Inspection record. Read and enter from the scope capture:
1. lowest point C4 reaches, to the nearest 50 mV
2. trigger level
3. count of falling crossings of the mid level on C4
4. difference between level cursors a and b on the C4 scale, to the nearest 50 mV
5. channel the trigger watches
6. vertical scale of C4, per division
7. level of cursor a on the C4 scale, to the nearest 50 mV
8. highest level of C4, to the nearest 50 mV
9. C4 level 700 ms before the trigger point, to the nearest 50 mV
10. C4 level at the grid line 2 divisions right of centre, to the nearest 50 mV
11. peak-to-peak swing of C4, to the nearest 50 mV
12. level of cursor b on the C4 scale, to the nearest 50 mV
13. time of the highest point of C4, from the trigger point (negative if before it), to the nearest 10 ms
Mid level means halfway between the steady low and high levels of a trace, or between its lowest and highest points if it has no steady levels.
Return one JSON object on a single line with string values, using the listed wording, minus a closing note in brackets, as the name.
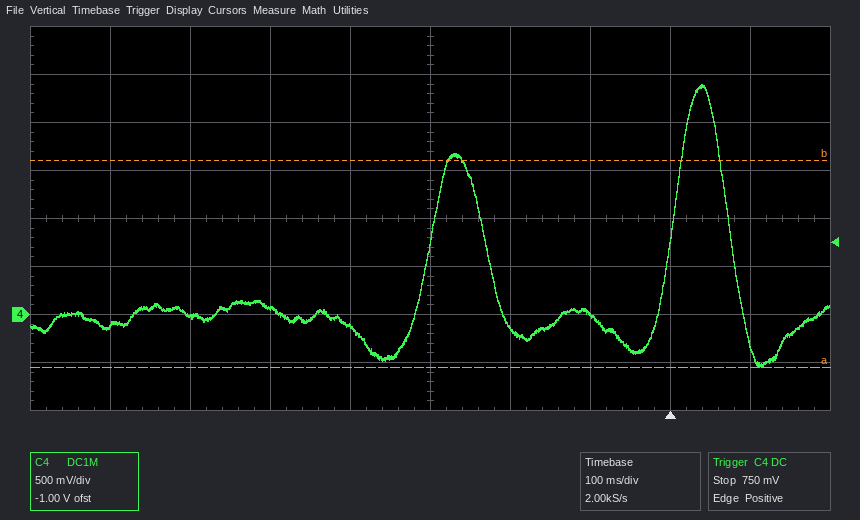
{"lowest point C4 reaches, to the nearest 50 mV": "-550 mV", "trigger level": "750 mV", "count of falling crossings of the mid level on C4": "2", "difference between level cursors a and b on the C4 scale, to the nearest 50 mV": "2.15 V", "channel the trigger watches": "C4", "vertical scale of C4, per division": "500 mV", "level of cursor a on the C4 scale, to the nearest 50 mV": "-550 mV", "highest level of C4, to the nearest 50 mV": "2.40 V", "C4 level 700 ms before the trigger point, to the nearest 50 mV": "-100 mV", "C4 level at the grid line 2 divisions right of centre, to the nearest 50 mV": "0 mV", "peak-to-peak swing of C4, to the nearest 50 mV": "2.95 V", "level of cursor b on the C4 scale, to the nearest 50 mV": "1.60 V", "time of the highest point of C4, from the trigger point (negative if before it), to the nearest 10 ms": "+40 ms"}
